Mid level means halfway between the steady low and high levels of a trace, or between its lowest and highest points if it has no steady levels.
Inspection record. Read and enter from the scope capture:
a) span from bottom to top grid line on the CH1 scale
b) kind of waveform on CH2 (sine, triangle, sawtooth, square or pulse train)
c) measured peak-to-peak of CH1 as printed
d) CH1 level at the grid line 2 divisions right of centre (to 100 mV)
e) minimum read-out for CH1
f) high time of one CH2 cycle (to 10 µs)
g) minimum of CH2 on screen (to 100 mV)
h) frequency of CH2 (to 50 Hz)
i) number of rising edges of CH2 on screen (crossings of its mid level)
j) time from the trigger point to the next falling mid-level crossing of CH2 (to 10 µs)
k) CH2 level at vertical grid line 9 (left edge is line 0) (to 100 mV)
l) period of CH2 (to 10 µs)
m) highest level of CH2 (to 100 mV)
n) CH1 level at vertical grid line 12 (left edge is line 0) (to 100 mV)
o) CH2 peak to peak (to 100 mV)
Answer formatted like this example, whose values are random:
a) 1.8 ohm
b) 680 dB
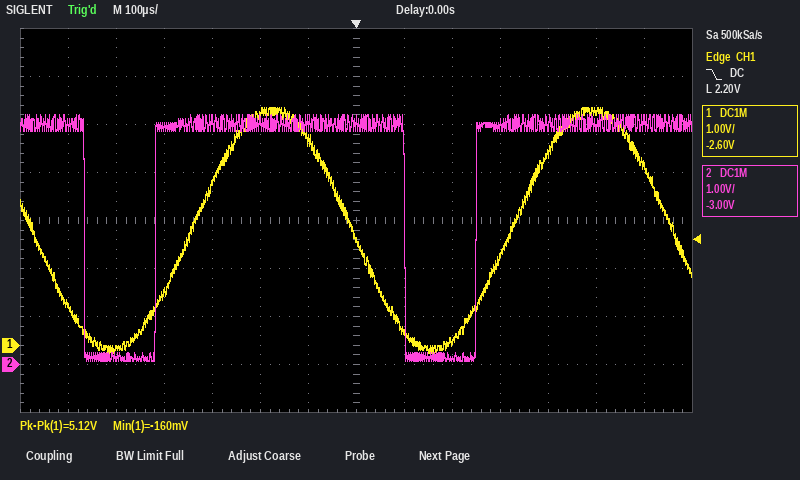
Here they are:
a) 8 V
b) pulse train
c) 5.12 V
d) 100 mV
e) -160 mV
f) 520 µs
g) 100 mV
h) 1.50 kHz
i) 2
j) 100 µs
k) 100 mV
l) 670 µs
m) 5.2 V
n) 4.9 V
o) 5.1 V
